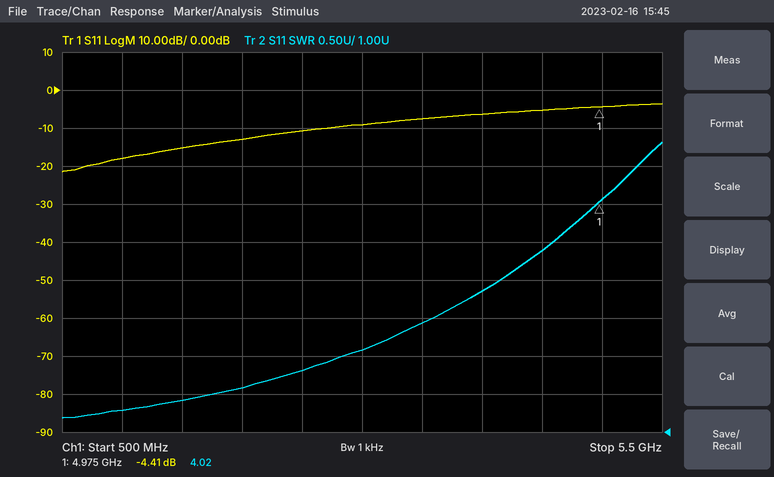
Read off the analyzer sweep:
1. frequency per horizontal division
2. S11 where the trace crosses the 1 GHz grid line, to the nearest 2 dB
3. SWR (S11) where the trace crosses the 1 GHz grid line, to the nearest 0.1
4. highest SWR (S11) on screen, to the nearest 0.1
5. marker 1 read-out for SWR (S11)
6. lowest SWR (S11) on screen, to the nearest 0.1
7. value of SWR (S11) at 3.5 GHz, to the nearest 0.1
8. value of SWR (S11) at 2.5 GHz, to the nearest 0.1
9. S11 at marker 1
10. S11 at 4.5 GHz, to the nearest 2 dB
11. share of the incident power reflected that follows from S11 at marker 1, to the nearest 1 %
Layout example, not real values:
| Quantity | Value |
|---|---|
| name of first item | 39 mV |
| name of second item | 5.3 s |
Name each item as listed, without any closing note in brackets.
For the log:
| Quantity | Value |
|---|---|
| frequency per horizontal division | 500 MHz |
| S11 where the trace crosses the 1 GHz grid line, to the nearest 2 dB | -18 dB |
| SWR (S11) where the trace crosses the 1 GHz grid line, to the nearest 0.1 | 1.3 |
| highest SWR (S11) on screen, to the nearest 0.1 | 4.8 |
| marker 1 read-out for SWR | 4.02 |
| lowest SWR (S11) on screen, to the nearest 0.1 | 1.2 |
| value of SWR (S11) at 3.5 GHz, to the nearest 0.1 | 2.4 |
| value of SWR (S11) at 2.5 GHz, to the nearest 0.1 | 1.8 |
| S11 at marker 1 | -4.41 dB |
| S11 at 4.5 GHz, to the nearest 2 dB | -6 dB |
| share of the incident power reflected that follows from S11 at marker 1, to the nearest 1 % | 36 % |
